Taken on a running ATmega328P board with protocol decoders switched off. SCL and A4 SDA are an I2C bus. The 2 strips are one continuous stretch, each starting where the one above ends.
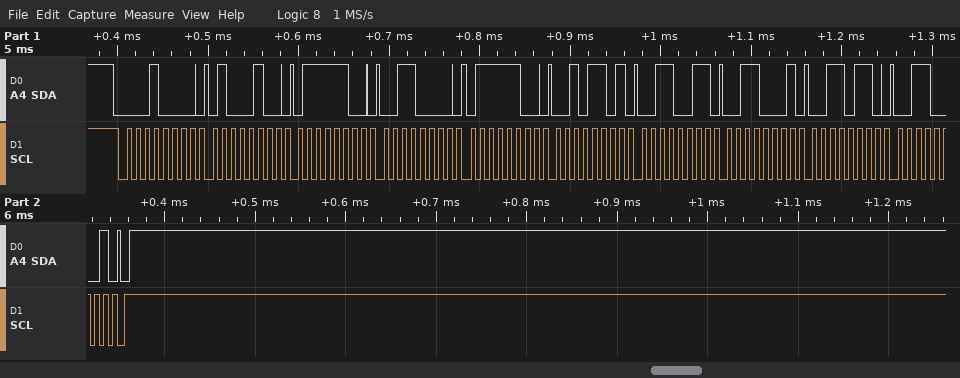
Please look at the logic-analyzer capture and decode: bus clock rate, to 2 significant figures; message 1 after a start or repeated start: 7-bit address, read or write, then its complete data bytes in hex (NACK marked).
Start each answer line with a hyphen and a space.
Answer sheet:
- 100 kHz
- 0x08 write: 44 7C 30 7C 2D 33 31 36 31
